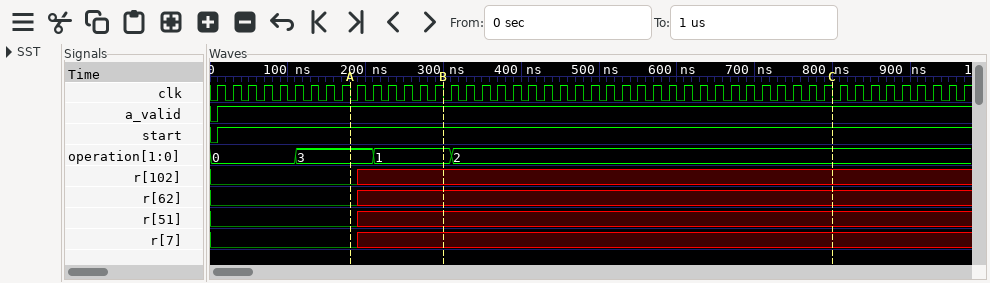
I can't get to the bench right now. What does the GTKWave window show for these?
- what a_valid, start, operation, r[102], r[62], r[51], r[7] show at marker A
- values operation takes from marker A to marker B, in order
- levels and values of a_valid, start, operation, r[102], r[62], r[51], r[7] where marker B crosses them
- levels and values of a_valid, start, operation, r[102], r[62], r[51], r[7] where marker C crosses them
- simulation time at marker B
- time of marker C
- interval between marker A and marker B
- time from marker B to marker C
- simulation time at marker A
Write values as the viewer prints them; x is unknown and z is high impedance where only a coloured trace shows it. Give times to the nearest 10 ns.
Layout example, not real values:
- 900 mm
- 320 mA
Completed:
- a_valid=1, start=1, operation=3, r[102]=0, r[62]=0, r[51]=0, r[7]=0
- 3, 1
- a_valid=1, start=1, operation=1, r[102]=x, r[62]=x, r[51]=x, r[7]=x
- a_valid=1, start=1, operation=2, r[102]=x, r[62]=x, r[51]=x, r[7]=x
- 300 ns
- 800 ns
- 120 ns
- 500 ns
- 180 ns
